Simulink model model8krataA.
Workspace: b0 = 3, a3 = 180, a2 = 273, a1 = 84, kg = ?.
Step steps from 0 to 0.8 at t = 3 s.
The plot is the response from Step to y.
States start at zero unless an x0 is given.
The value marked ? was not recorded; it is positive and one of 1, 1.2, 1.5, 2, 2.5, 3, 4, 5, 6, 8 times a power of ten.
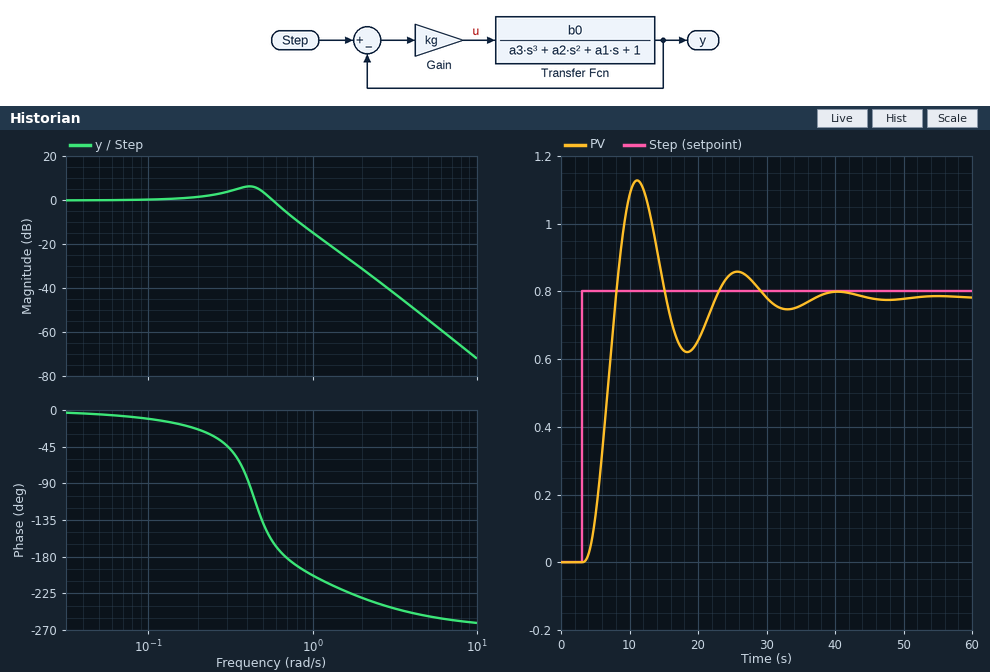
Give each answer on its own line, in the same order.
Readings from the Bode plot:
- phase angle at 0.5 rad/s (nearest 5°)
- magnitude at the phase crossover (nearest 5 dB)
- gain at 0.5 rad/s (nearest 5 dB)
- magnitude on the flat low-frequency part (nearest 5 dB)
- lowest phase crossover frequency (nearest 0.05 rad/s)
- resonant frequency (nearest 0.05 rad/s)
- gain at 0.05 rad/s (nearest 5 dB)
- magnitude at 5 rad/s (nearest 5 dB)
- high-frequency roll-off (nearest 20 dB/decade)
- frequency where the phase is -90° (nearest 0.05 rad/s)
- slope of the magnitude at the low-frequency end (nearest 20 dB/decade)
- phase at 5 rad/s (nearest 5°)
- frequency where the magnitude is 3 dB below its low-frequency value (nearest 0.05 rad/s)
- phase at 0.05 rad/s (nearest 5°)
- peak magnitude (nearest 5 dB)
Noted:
-140°
-5 dB
5 dB
0 dB
0.70 rad/s
0.40 rad/s
0 dB
-55 dB
-60 dB/decade
0.40 rad/s
0 dB/decade
-255°
0.65 rad/s
-5°
5 dB
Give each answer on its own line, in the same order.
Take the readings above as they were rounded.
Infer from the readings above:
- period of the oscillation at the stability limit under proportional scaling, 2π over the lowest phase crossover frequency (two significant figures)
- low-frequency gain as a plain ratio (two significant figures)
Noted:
9.0 s
1.0
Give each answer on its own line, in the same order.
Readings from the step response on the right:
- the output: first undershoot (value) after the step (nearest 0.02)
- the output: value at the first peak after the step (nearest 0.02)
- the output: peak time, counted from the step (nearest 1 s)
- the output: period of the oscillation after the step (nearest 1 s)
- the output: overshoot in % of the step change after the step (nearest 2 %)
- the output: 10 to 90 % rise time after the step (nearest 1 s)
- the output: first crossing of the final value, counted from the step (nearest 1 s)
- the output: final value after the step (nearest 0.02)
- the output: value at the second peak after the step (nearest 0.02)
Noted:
0.62
1.12
8 s
15 s
44 %
3 s
5 s
0.78
0.86
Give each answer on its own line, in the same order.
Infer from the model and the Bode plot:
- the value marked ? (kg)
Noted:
15
